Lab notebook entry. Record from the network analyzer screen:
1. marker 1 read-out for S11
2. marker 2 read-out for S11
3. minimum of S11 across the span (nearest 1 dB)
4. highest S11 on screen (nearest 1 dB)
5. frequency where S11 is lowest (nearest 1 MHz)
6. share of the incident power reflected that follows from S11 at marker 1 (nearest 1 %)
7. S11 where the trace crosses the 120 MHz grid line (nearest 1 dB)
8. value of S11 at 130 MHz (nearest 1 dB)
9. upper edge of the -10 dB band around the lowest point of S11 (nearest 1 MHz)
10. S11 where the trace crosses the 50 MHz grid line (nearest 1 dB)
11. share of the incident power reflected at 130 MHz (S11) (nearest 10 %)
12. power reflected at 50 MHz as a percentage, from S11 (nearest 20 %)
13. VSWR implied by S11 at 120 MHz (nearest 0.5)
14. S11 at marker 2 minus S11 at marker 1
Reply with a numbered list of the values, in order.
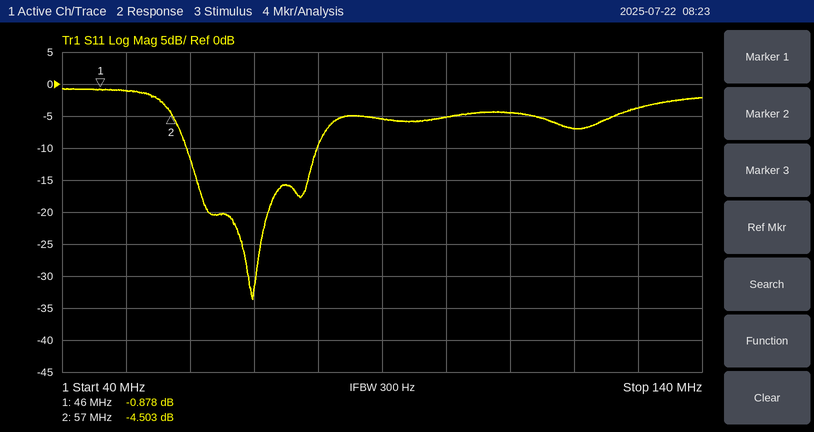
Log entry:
1. -0.878 dB
2. -4.503 dB
3. -34 dB
4. -1 dB
5. 70 MHz
6. 82 %
7. -7 dB
8. -4 dB
9. 80 MHz
10. -1 dB
11. 40 %
12. 80 %
13. 2.5
14. -3.625 dB
